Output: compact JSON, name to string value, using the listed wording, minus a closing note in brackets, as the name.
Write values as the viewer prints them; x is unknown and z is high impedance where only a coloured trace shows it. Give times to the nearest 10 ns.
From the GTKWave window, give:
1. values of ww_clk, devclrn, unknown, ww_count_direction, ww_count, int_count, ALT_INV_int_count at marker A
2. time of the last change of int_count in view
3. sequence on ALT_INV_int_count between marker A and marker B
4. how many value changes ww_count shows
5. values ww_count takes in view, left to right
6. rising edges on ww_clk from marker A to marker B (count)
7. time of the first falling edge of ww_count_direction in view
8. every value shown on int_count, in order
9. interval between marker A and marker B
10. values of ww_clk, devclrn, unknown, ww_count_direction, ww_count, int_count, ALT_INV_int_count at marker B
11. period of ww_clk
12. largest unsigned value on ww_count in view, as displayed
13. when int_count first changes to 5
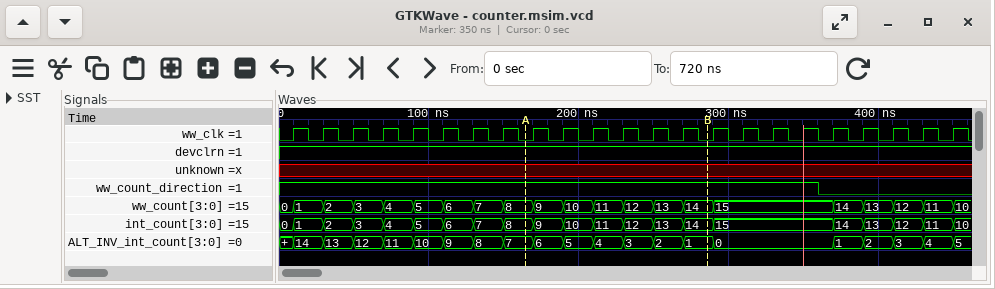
{"values of ww_clk, devclrn, unknown, ww_count_direction, ww_count, int_count, ALT_INV_int_count at marker A": "ww_clk=0, devclrn=1, unknown=x, ww_count_direction=1, ww_count=8, int_count=8, ALT_INV_int_count=7", "time of the last change of int_count in view": "450 ns", "sequence on ALT_INV_int_count between marker A and marker B": "7, 6, 5, 4, 3, 2, 1", "how many value changes ww_count shows": "20", "values ww_count takes in view, left to right": "0, 1, 2, 3, 4, 5, 6, 7, 8, 9, 10, 11, 12, 13, 14, 15, 14, 13, 12, 11, 10", "rising edges on ww_clk from marker A to marker B": "6", "time of the first falling edge of ww_count_direction in view": "360 ns", "every value shown on int_count, in order": "0, 1, 2, 3, 4, 5, 6, 7, 8, 9, 10, 11, 12, 13, 14, 15, 14, 13, 12, 11, 10", "interval between marker A and marker B": "120 ns", "values of ww_clk, devclrn, unknown, ww_count_direction, ww_count, int_count, ALT_INV_int_count at marker B": "ww_clk=0, devclrn=1, unknown=x, ww_count_direction=1, ww_count=14, int_count=14, ALT_INV_int_count=1", "period of ww_clk": "20 ns", "largest unsigned value on ww_count in view, as displayed": "15", "when int_count first changes to 5": "90 ns"}
